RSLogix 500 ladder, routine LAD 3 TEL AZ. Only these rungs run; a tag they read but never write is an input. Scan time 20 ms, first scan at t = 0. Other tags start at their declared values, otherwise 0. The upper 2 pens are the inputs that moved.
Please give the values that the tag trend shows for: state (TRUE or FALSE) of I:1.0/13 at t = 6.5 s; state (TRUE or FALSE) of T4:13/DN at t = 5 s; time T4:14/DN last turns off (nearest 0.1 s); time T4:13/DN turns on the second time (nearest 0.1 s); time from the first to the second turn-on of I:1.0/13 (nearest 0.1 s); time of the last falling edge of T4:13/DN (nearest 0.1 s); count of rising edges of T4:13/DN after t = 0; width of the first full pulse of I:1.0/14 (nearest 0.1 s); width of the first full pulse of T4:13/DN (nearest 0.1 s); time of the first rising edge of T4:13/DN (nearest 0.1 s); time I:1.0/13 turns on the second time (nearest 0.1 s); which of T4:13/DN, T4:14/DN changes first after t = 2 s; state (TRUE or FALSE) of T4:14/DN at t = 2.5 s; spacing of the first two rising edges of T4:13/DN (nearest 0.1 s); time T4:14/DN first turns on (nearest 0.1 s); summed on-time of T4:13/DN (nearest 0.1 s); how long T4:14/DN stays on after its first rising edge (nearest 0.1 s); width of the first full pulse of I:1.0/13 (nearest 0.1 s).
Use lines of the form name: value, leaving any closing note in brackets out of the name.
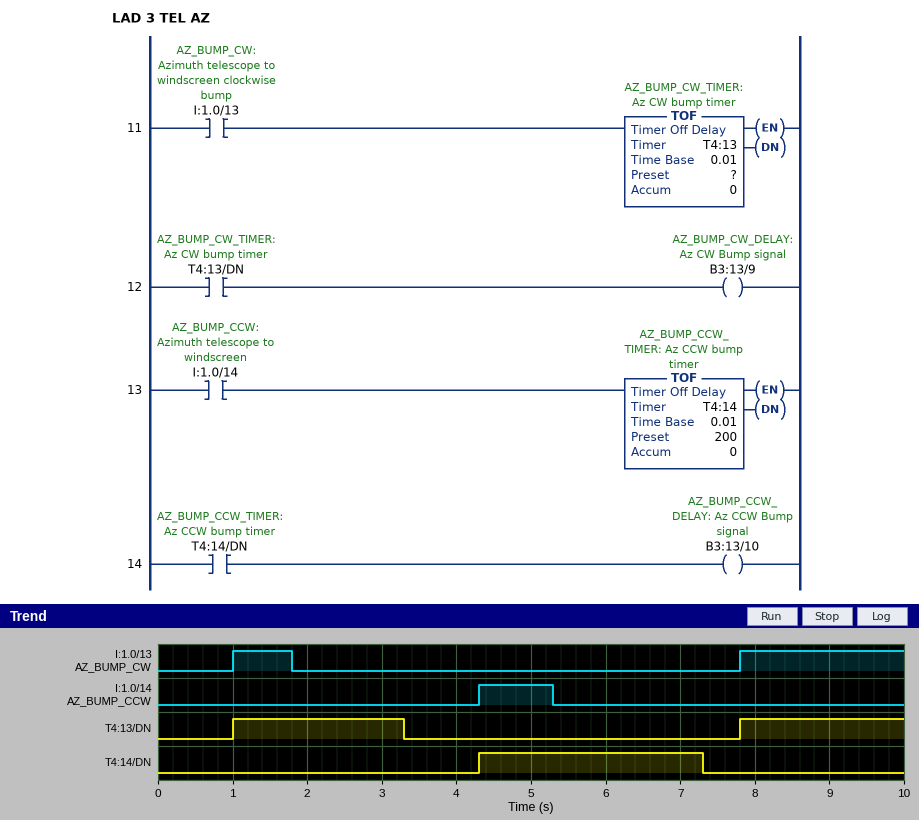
state (TRUE or FALSE) of I:1.0/13 at t = 6.5 s: FALSE
state (TRUE or FALSE) of T4:13/DN at t = 5 s: FALSE
time T4:14/DN last turns off: 7.3 s
time T4:13/DN turns on the second time: 7.8 s
time from the first to the second turn-on of I:1.0/13: 6.8 s
time of the last falling edge of T4:13/DN: 3.3 s
count of rising edges of T4:13/DN after t = 0: 2
width of the first full pulse of I:1.0/14: 1.0 s
width of the first full pulse of T4:13/DN: 2.3 s
time of the first rising edge of T4:13/DN: 1.0 s
time I:1.0/13 turns on the second time: 7.8 s
which of T4:13/DN, T4:14/DN changes first after t = 2 s: T4:13/DN
state (TRUE or FALSE) of T4:14/DN at t = 2.5 s: FALSE
spacing of the first two rising edges of T4:13/DN: 6.8 s
time T4:14/DN first turns on: 4.3 s
summed on-time of T4:13/DN: 4.5 s
how long T4:14/DN stays on after its first rising edge: 3.0 s
width of the first full pulse of I:1.0/13: 0.8 s
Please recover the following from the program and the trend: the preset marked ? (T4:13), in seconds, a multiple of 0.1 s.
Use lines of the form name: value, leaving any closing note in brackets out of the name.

the preset marked ? (T4:13), in seconds, a multiple of 0.1 s: 1.5 s
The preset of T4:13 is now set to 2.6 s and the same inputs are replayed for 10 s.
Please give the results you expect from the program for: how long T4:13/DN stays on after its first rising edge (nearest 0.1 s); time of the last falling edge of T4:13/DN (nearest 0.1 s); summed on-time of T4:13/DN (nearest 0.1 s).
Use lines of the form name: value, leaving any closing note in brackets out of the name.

how long T4:13/DN stays on after its first rising edge: 3.4 s
time of the last falling edge of T4:13/DN: 4.4 s
summed on-time of T4:13/DN: 5.6 s
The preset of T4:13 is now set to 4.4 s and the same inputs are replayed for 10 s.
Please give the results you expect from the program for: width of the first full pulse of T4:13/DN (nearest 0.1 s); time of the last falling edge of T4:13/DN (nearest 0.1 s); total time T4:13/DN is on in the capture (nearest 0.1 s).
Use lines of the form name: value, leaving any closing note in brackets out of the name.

width of the first full pulse of T4:13/DN: 5.2 s
time of the last falling edge of T4:13/DN: 6.2 s
total time T4:13/DN is on in the capture: 7.4 s
